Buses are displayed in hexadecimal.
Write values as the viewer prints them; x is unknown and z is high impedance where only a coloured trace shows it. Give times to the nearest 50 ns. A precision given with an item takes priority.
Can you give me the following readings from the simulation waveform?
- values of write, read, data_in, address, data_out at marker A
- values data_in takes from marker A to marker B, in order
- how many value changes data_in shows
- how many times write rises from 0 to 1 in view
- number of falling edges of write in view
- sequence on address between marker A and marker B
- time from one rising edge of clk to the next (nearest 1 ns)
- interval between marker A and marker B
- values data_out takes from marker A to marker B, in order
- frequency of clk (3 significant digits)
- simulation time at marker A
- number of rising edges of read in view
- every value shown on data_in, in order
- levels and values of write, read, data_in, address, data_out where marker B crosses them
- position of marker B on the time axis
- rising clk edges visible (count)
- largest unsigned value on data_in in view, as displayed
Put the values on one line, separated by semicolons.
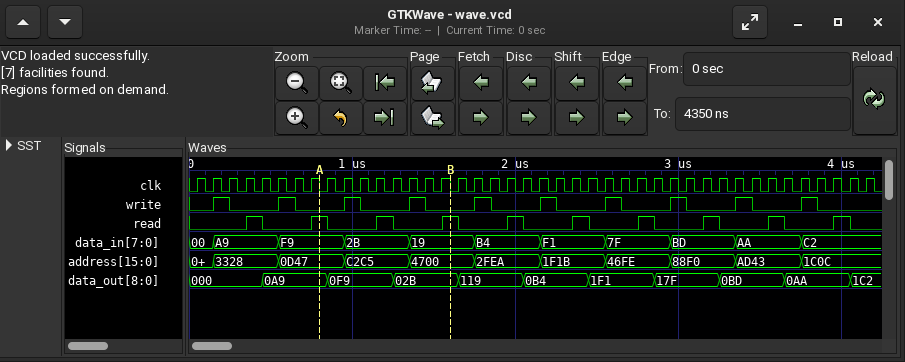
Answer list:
write=0, read=1, data_in=F9, address=0D47, data_out=0A9; F9, 2B, 19; 10; 10; 10; 0D47, C2C5, 4700; 100 ns; 800 ns; 0A9, 0F9, 02B; 10.0 MHz; 800 ns; 10; 00, A9, F9, 2B, 19, B4, F1, 7F, BD, AA, C2; write=0, read=1, data_in=19, address=4700, data_out=02B; 1600 ns; 42; F9
